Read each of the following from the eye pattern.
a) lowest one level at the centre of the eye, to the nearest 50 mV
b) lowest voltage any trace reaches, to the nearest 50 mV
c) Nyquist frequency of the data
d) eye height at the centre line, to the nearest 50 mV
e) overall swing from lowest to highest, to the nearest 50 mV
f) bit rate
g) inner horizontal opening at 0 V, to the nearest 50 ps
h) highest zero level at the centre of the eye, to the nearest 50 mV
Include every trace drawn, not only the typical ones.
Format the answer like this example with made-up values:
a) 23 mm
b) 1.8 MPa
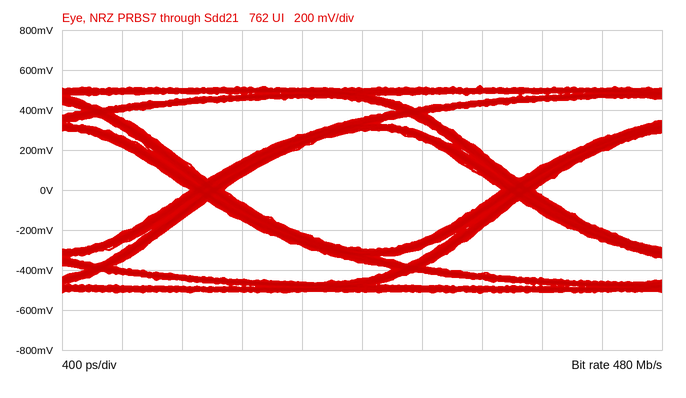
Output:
a) 300 mV
b) -500 mV
c) 240 MHz
d) 600 mV
e) 1.05 V
f) 480 Mb/s
g) 1.85 ns
h) -300 mV
